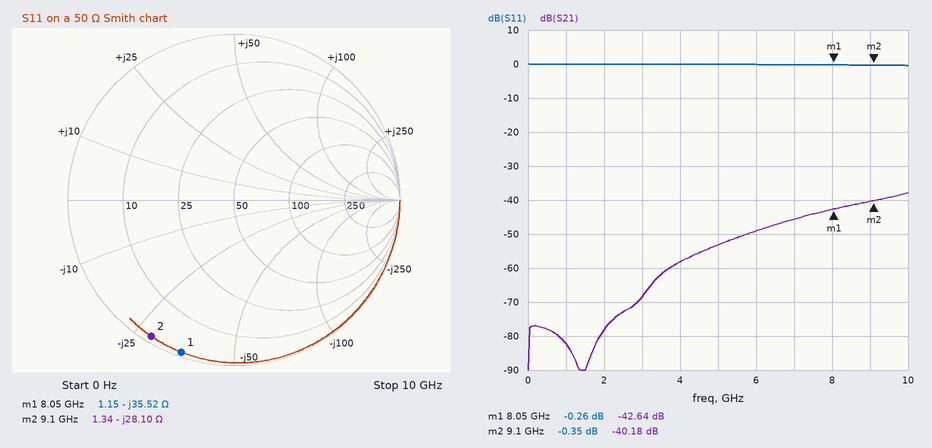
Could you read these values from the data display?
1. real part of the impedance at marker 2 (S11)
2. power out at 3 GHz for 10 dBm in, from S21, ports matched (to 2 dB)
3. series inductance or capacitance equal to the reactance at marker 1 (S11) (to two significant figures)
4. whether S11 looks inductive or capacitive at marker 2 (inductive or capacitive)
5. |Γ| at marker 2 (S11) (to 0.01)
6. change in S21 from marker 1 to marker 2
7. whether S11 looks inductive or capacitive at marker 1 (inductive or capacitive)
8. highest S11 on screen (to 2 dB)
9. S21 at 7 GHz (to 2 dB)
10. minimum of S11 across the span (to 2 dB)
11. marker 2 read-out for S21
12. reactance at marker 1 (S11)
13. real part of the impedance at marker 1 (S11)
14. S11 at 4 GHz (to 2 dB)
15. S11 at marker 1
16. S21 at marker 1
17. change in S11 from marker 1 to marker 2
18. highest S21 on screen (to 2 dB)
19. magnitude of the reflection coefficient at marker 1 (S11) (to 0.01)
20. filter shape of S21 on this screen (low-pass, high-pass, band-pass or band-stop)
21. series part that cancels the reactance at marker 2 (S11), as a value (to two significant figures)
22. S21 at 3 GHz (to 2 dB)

1.34 Ω
-58 dBm
560 fF
capacitive
0.96
2.46 dB
capacitive
0 dB
-46 dB
0 dB
-40.18 dB
-35.52 Ω
1.15 Ω
0 dB
-0.26 dB
-42.64 dB
-0.09 dB
-38 dB
0.97
high-pass
490 pH
-68 dB
